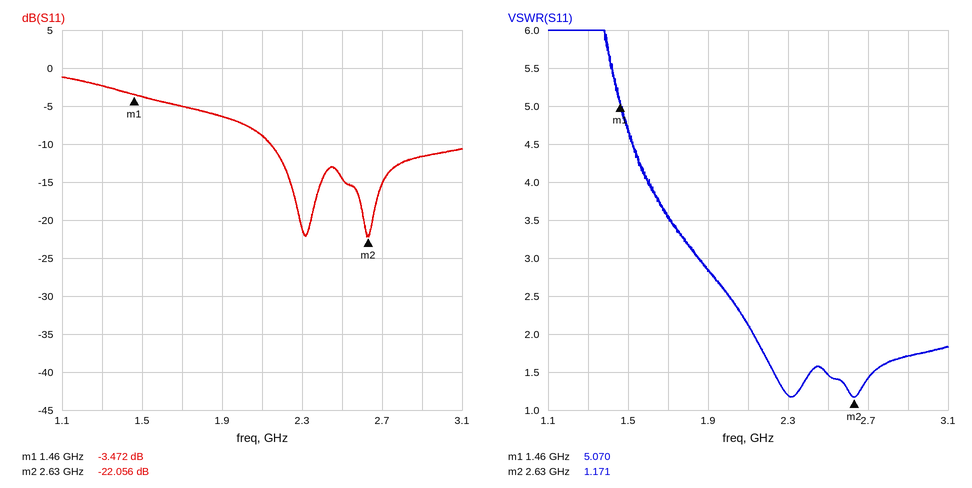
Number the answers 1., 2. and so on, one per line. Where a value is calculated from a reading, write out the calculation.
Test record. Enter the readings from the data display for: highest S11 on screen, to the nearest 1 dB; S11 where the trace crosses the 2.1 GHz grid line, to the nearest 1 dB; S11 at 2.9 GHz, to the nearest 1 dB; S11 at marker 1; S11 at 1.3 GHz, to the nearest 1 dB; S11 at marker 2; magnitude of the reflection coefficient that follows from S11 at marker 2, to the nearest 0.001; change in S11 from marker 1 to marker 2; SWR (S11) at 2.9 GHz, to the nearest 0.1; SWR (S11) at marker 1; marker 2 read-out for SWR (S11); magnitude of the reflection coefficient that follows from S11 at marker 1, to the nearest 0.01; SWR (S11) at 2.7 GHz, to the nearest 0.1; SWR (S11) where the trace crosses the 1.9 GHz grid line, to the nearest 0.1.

1. -1 dB
2. -9 dB
3. -12 dB
4. -3.472 dB
5. -2 dB
6. -22.056 dB
7. 10^(-22.056/20) ≈ 0.079
8. -22.056 − (-3.472) = -18.584 dB
9. 1.7
10. 5.070
11. 1.171
12. 10^(-3.472/20) ≈ 0.67
13. 1.4
14. 2.8
